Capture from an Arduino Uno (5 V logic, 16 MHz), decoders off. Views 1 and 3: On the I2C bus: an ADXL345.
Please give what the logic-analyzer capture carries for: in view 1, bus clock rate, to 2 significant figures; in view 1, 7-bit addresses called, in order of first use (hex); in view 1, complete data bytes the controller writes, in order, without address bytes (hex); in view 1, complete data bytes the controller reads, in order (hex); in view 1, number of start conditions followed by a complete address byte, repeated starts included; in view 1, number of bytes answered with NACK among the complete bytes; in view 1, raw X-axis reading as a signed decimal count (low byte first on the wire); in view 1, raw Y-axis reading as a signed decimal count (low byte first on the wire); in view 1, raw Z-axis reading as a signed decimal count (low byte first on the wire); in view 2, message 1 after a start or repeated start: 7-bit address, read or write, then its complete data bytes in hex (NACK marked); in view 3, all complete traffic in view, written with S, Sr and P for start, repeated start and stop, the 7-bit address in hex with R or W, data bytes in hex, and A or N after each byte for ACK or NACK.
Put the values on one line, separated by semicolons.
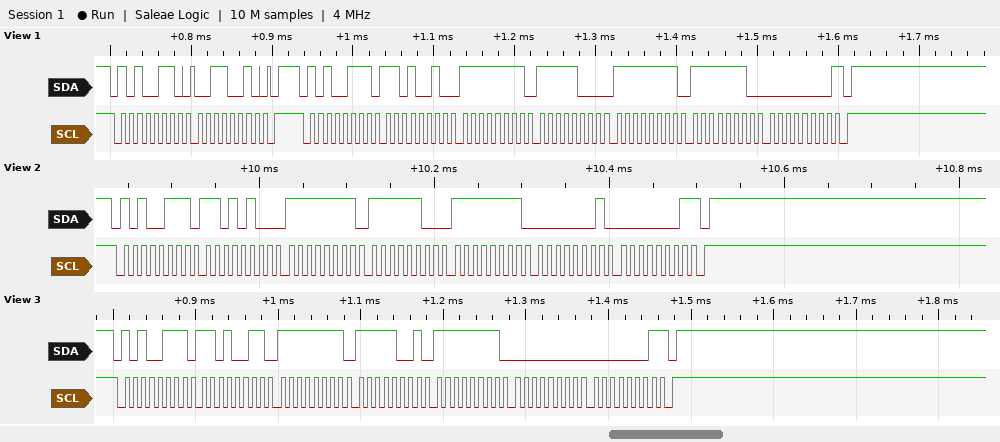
100 kHz; 0x53; 32; D2 FF F8 FF FE 00; 2; 1; -46; -8; 254; 0x53 read: D4 FF FC FF 01 01 NACK; S 53R A D3 A FF A F9 A FF A 00 A 01 N P
